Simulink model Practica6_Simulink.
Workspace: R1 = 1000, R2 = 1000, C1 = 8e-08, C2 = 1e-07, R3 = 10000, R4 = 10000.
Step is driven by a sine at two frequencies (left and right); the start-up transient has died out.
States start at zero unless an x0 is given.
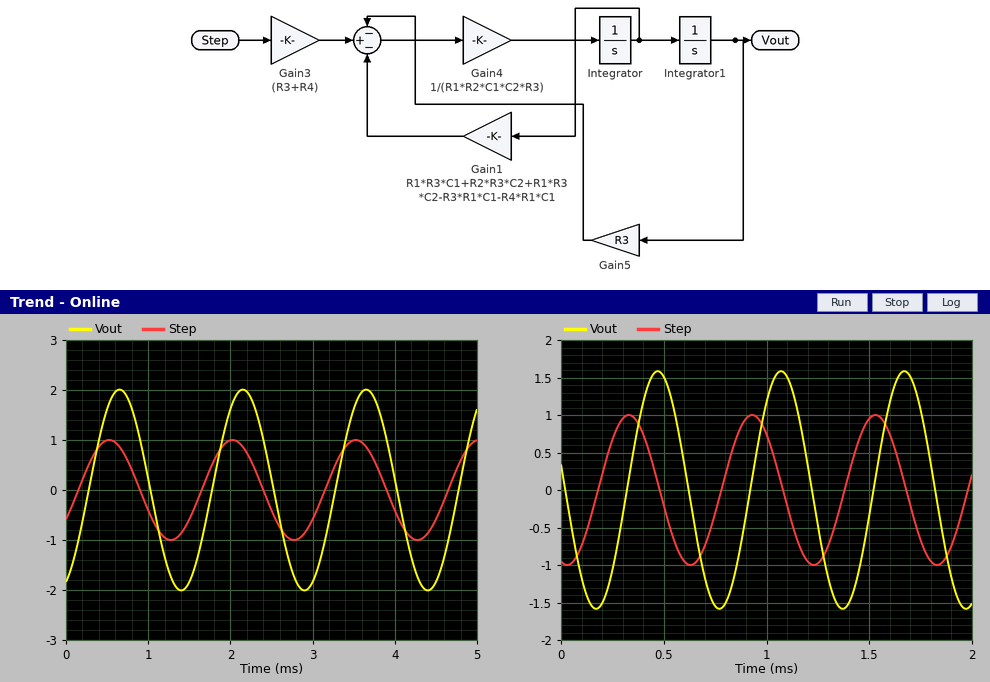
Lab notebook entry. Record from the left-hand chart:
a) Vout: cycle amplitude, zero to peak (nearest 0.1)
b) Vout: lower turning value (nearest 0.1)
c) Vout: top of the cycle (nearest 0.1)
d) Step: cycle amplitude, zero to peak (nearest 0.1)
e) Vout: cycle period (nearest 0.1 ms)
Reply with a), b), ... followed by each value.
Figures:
a) 2.0
b) -2.0
c) 2.0
d) 1.0
e) 1.5 ms
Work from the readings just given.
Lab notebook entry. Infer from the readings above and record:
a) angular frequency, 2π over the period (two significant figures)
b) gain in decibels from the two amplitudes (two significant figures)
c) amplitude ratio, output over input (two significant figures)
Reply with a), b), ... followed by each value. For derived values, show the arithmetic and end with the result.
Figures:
a) 2π / 1.5 = 4.2 rad/ms
b) 20 log10(2 / 1) = 6.0 dB
c) 2 / 1 = 2.0
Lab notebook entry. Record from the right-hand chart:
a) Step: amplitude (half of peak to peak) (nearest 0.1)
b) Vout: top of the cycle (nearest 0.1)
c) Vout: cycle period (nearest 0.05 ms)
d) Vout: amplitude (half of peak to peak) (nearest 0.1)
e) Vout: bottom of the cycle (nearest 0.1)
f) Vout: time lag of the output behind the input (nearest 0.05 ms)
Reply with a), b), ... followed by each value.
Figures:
a) 1.0
b) 1.6
c) 0.60 ms
d) 1.6
e) -1.6
f) 0.15 ms
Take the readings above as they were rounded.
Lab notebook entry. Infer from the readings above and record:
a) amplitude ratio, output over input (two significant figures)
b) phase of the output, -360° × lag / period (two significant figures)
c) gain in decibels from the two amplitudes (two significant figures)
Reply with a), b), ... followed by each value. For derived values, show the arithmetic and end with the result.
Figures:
a) 1.6 / 1 = 1.6
b) -360 × 0.15 / 0.6 = -90°
c) 20 log10(1.6 / 1) = 4.1 dB
